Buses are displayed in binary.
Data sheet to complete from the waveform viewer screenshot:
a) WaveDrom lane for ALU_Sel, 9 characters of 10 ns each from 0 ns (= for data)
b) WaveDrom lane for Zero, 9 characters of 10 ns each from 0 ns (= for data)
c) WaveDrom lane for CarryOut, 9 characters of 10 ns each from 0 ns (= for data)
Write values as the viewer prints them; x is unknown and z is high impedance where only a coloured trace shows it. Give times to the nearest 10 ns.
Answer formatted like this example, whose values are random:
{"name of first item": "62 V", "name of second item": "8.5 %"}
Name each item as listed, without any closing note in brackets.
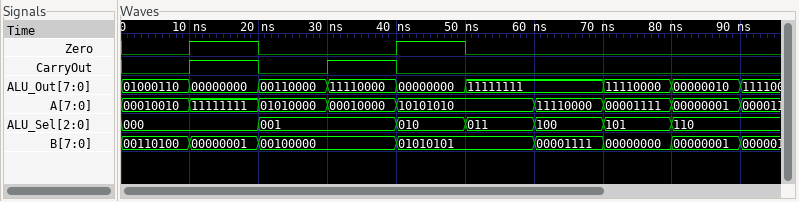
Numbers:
{"WaveDrom lane for ALU_Sel, 9 characters of 10 ns each from 0 ns": "{name: 'ALU_Sel', wave: '=.=.=====', data: '000 001 010 011 100 101 110'}", "WaveDrom lane for Zero, 9 characters of 10 ns each from 0 ns": "{name: 'Zero', wave: '010.10...'}", "WaveDrom lane for CarryOut, 9 characters of 10 ns each from 0 ns": "{name: 'CarryOut', wave: '01010....'}"}
